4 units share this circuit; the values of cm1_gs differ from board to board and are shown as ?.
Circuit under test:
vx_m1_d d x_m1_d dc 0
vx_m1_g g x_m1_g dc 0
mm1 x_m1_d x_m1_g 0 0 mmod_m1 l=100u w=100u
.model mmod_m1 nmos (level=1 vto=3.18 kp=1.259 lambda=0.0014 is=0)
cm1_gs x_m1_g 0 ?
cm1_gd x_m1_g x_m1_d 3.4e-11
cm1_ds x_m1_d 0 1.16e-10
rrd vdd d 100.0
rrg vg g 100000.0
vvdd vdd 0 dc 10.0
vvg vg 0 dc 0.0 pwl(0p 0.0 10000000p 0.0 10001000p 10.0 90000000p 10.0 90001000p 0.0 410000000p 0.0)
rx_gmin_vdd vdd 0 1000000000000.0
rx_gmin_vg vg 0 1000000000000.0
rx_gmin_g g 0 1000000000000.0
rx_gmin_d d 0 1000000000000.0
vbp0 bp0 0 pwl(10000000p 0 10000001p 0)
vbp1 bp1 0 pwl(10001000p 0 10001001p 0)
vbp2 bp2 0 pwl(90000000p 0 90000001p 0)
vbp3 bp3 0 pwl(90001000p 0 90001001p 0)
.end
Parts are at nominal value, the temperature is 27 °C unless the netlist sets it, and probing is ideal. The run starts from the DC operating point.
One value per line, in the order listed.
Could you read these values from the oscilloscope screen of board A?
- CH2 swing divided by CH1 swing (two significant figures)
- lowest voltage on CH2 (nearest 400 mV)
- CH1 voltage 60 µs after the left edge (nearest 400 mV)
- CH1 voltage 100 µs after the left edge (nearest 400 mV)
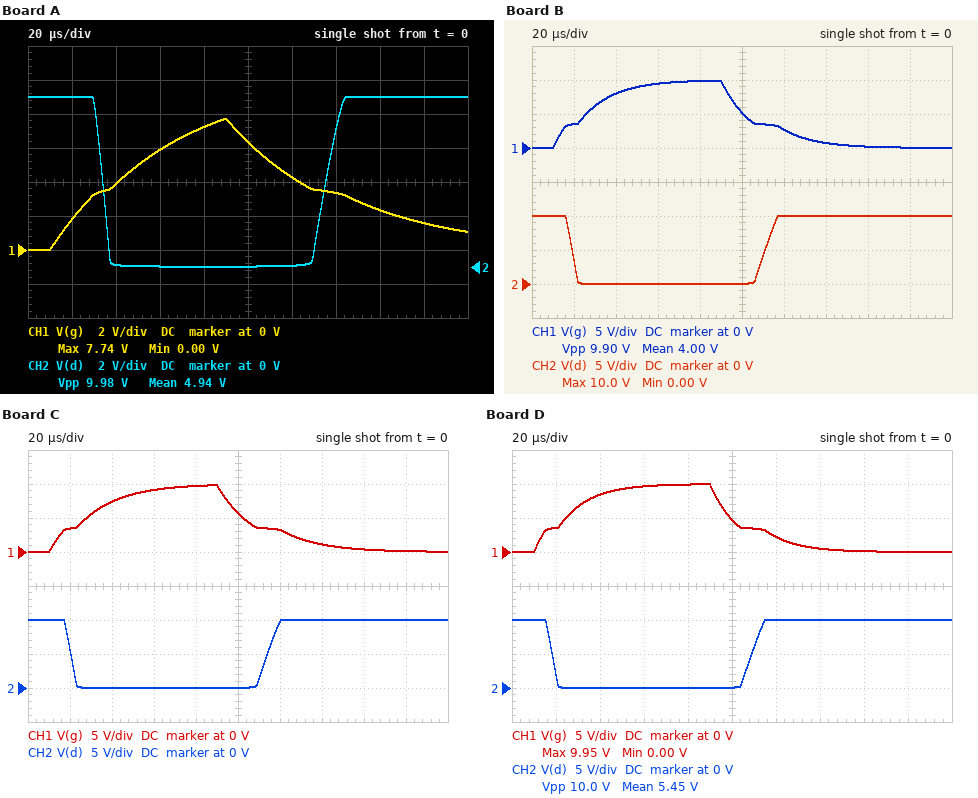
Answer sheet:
1.3
0 V
6.0 V
6.4 V
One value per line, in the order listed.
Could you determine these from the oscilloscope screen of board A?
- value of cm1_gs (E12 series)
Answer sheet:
470 pF
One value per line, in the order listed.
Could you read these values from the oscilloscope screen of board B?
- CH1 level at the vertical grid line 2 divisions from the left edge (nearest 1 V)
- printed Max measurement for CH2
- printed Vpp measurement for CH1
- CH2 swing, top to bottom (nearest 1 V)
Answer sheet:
8 V
10.0 V
9.90 V
10 V
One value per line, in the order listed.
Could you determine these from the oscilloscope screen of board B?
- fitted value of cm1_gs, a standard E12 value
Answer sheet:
120 pF
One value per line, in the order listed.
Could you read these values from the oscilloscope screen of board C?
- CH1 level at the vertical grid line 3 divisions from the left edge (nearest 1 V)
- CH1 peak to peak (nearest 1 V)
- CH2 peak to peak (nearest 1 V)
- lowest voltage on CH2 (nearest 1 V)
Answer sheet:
9 V
10 V
10 V
0 V
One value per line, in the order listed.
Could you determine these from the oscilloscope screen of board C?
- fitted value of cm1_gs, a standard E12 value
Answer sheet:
150 pF
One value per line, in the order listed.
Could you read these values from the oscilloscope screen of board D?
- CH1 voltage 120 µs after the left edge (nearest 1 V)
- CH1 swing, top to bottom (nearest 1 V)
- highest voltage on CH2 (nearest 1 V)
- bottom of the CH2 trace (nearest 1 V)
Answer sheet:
2 V
10 V
10 V
0 V
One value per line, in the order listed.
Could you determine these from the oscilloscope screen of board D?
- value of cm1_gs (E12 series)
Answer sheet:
100 pF
